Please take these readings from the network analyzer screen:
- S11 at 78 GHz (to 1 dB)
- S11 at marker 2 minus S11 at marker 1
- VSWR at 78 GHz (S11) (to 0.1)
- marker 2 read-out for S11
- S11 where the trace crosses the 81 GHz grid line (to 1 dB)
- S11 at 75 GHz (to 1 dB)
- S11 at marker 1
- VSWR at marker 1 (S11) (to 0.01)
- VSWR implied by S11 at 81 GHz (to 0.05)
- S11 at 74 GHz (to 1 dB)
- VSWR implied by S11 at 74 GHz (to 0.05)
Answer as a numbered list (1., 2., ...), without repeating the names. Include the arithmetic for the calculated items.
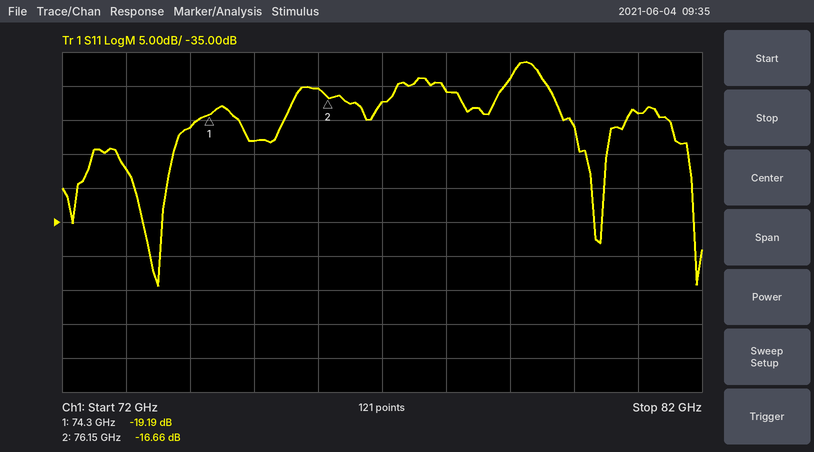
1. -16 dB
2. -16.66 − (-19.19) = 2.53 dB
3. |Γ| = 10^(-16/20) = 0.1585; VSWR = (1 + 0.1585)/(1 − 0.1585) ≈ 1.4
4. -16.66 dB
5. -19 dB
6. -23 dB
7. -19.19 dB
8. (1 + 0.1098)/(1 − 0.1098) ≈ 1.25
9. |Γ| = 10^(-19/20) = 0.1122; VSWR = (1 + 0.1122)/(1 − 0.1122) ≈ 1.25
10. -21 dB
11. |Γ| = 10^(-21/20) = 0.0891; VSWR = (1 + 0.0891)/(1 − 0.0891) ≈ 1.20
